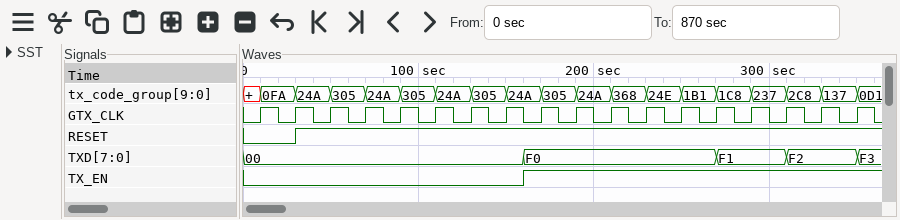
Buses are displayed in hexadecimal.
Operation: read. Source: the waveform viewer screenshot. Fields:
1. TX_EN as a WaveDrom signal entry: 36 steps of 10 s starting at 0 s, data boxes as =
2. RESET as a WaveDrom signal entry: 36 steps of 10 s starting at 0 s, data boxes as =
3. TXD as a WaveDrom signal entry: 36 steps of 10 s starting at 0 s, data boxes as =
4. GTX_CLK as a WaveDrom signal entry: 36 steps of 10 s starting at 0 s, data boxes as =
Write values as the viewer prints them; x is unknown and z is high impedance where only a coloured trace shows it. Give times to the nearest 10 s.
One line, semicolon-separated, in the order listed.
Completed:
{name: 'TX_EN', wave: '0...............1...................'}; {name: 'RESET', wave: '0..1................................'}; {name: 'TXD', wave: '=...............=..........=...=...=', data: '00 F0 F1 F2 F3'}; {name: 'GTX_CLK', wave: '010101010101010101010101010101010101'}
